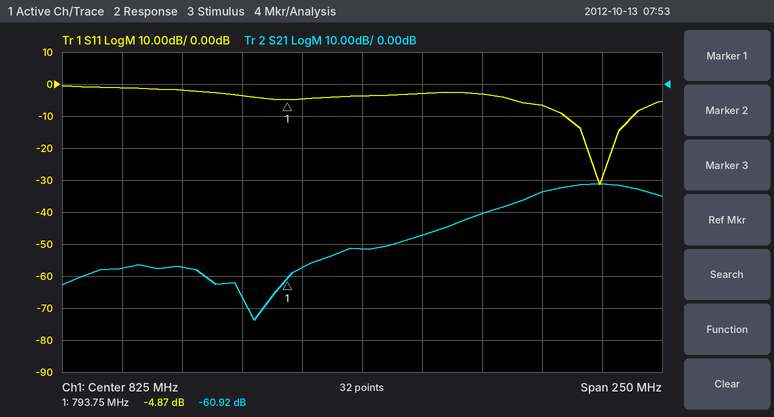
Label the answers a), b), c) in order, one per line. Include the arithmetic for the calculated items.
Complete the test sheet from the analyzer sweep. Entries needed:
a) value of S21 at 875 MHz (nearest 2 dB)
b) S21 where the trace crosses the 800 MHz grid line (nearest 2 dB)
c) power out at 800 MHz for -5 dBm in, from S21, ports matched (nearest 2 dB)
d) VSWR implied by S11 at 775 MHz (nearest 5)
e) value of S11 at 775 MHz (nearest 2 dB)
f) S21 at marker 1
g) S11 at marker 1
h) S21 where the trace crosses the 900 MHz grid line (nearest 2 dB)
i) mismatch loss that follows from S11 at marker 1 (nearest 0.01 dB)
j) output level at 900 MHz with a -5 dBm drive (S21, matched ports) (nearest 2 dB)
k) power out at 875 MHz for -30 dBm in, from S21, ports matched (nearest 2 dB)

a) -40 dB
b) -58 dB
c) -5 dBm + (-58 dB) = -62 dBm
d) |Γ| = 10^(-4/20) = 0.6310; VSWR = (1 + 0.6310)/(1 − 0.6310) ≈ 4.42, so 5 to the nearest 5
e) -4 dB
f) -60.92 dB
g) -4.87 dB
h) -34 dB
i) −10 log10(1 − 10^(-4.87/10)) ≈ 1.71 dB
j) -5 dBm + (-34 dB) = -38 dBm
k) -30 dBm + (-40 dB) = -70 dBm
